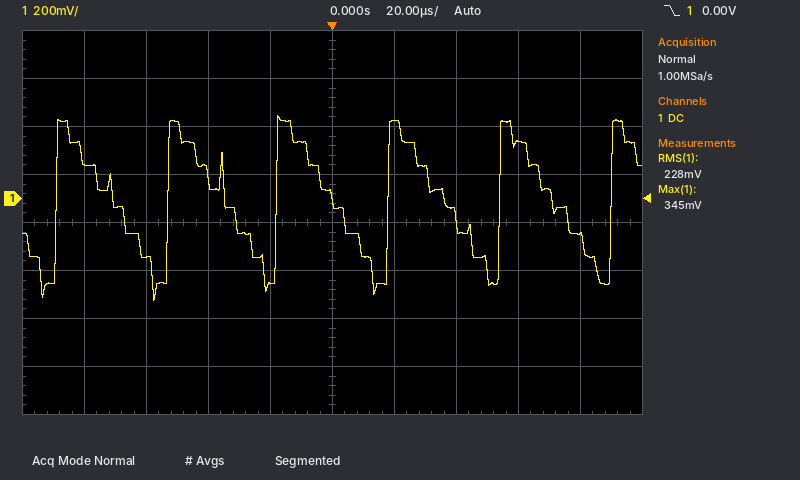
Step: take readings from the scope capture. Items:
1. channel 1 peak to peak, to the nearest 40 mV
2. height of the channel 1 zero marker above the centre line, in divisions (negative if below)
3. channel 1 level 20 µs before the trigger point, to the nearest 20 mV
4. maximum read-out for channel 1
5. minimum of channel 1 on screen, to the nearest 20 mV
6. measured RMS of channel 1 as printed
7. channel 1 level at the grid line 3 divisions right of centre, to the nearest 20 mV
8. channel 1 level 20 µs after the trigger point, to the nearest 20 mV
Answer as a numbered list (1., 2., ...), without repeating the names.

1. 760 mV
2. +0.5 div
3. -360 mV
4. 345 mV
5. -420 mV
6. 228 mV
7. 240 mV
8. 320 mV
